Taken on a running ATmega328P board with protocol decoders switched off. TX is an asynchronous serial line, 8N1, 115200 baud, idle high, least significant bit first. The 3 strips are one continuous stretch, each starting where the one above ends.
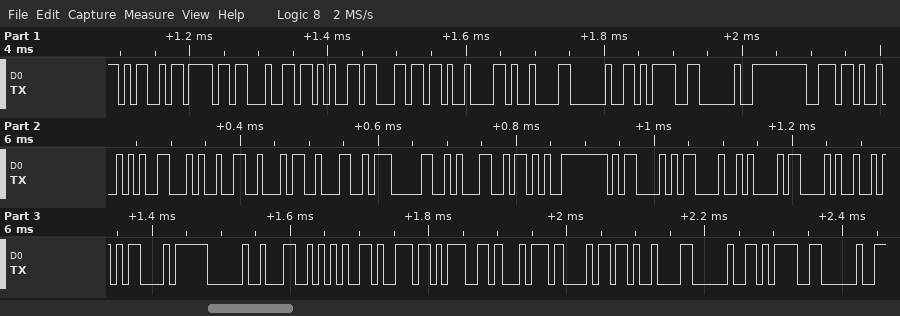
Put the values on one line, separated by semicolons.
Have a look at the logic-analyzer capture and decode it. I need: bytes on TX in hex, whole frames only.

0x4D 0x6F 0x64 0x65 0x6C 0x09 0x09 0x20 0x3D 0x20 0x6E 0x52 0x46 0x32 0x34 0x4C 0x30 0x31 0x2B 0x0D 0x0D 0x0A 0x43 0x52 0x43 0x20 0x4C 0x65 0x6E 0x67 0x74 0x68 0x09 0x20 0x3D 0x20
